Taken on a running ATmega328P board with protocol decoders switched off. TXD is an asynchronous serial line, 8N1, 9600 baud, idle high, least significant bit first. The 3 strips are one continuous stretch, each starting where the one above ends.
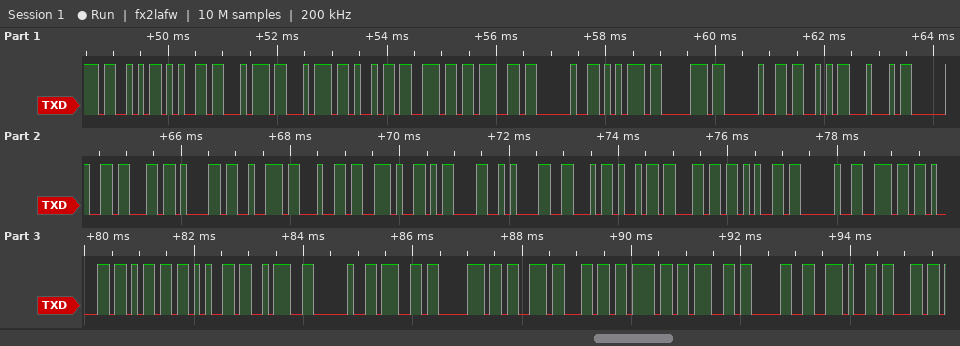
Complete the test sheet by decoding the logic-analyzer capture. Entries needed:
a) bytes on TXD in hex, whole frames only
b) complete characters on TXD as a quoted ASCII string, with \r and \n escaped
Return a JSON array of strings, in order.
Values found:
["53 65 74 74 69 6E 67 20 75 70 20 53 44 20 63 61 72 64 2E 0D 0A 46 69 6C 65 20 6E 61 6D 65 3A 20 67 70 73 6C 6F 67 30 2E 63", "\"Setting up SD card.\\r\\nFile name: gpslog0.c\""]
